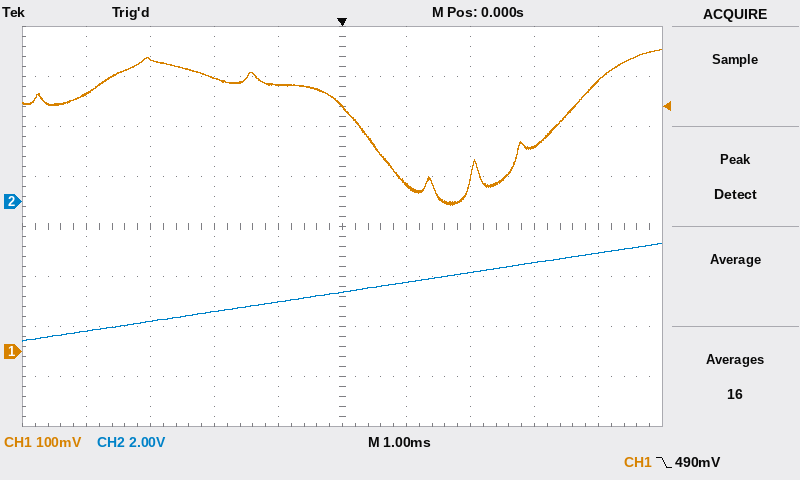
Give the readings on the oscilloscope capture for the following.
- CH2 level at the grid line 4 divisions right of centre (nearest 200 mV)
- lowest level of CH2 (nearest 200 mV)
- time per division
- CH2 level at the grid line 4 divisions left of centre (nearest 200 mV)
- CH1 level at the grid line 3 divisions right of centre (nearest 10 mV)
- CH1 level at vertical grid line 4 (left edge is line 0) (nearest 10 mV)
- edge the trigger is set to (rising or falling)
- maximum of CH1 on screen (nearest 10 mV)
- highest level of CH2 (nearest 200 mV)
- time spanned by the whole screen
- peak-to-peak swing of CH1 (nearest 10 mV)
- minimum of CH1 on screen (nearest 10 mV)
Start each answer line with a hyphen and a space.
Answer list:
- -2.0 V
- -5.6 V
- 1 ms
- -5.2 V
- 410 mV
- 530 mV
- falling
- 600 mV
- -1.6 V
- 10 ms
- 310 mV
- 290 mV
